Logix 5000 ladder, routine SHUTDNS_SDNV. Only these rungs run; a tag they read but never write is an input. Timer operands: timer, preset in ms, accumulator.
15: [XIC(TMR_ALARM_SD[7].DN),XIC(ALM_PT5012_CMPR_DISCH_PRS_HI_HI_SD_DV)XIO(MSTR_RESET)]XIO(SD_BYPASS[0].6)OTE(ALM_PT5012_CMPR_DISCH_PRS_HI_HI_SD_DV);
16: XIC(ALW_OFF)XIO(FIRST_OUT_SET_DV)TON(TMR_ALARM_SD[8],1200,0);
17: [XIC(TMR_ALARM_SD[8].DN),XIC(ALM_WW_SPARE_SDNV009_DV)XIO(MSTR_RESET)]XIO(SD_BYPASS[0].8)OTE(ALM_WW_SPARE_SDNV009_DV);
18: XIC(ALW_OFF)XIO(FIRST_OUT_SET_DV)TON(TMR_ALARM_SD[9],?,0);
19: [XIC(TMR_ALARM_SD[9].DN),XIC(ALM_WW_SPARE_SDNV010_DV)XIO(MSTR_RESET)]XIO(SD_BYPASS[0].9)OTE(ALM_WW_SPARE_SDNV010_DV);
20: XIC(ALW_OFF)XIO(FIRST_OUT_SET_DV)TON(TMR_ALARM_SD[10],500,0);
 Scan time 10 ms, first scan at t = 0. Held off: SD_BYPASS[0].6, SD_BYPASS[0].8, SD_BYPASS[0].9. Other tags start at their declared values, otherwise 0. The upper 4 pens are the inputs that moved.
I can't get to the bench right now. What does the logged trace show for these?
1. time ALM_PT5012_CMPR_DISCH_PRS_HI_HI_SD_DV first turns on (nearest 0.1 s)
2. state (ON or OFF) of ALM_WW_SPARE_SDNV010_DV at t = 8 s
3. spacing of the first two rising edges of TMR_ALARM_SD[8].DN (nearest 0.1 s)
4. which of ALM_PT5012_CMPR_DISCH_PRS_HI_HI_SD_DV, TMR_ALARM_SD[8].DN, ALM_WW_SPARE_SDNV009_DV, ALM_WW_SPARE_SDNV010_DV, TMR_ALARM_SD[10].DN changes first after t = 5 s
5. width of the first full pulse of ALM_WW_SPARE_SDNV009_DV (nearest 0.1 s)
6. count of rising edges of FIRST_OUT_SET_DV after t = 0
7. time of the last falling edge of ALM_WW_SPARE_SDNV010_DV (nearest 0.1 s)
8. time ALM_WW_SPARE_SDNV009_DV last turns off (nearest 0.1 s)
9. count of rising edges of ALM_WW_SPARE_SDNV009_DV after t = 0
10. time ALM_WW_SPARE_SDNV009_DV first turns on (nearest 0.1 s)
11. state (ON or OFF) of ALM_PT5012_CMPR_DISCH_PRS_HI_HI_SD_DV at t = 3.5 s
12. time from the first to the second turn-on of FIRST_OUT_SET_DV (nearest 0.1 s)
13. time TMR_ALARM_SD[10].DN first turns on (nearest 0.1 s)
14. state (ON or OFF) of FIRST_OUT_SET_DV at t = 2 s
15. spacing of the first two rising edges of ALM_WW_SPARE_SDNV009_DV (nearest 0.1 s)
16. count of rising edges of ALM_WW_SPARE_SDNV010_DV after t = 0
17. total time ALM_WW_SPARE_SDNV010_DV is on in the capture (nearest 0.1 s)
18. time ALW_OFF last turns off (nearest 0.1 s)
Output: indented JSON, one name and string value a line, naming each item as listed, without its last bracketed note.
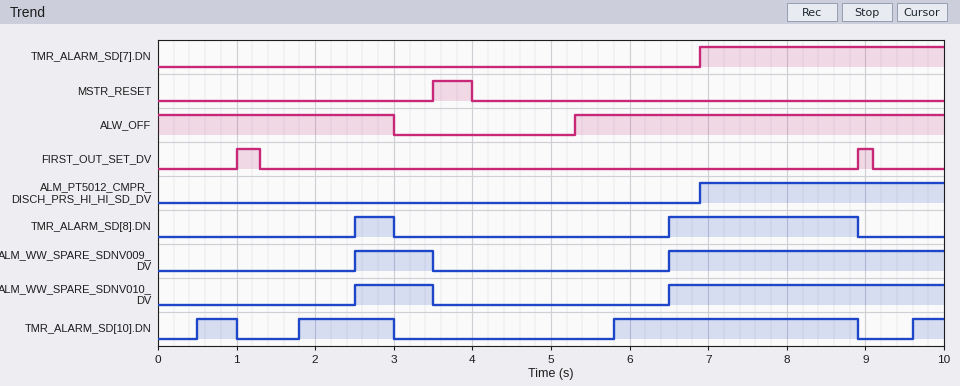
{
  "time ALM_PT5012_CMPR_DISCH_PRS_HI_HI_SD_DV first turns on": "6.9 s",
  "state (ON or OFF) of ALM_WW_SPARE_SDNV010_DV at t = 8 s": "ON",
  "spacing of the first two rising edges of TMR_ALARM_SD[8].DN": "4.0 s",
  "which of ALM_PT5012_CMPR_DISCH_PRS_HI_HI_SD_DV, TMR_ALARM_SD[8].DN, ALM_WW_SPARE_SDNV009_DV, ALM_WW_SPARE_SDNV010_DV, TMR_ALARM_SD[10].DN changes first after t = 5 s": "TMR_ALARM_SD[10].DN",
  "width of the first full pulse of ALM_WW_SPARE_SDNV009_DV": "1.0 s",
  "count of rising edges of FIRST_OUT_SET_DV after t = 0": "2",
  "time of the last falling edge of ALM_WW_SPARE_SDNV010_DV": "3.5 s",
  "time ALM_WW_SPARE_SDNV009_DV last turns off": "3.5 s",
  "count of rising edges of ALM_WW_SPARE_SDNV009_DV after t = 0": "2",
  "time ALM_WW_SPARE_SDNV009_DV first turns on": "2.5 s",
  "state (ON or OFF) of ALM_PT5012_CMPR_DISCH_PRS_HI_HI_SD_DV at t = 3.5 s": "OFF",
  "time from the first to the second turn-on of FIRST_OUT_SET_DV": "7.9 s",
  "time TMR_ALARM_SD[10].DN first turns on": "0.5 s",
  "state (ON or OFF) of FIRST_OUT_SET_DV at t = 2 s": "OFF",
  "spacing of the first two rising edges of ALM_WW_SPARE_SDNV009_DV": "4.0 s",
  "count of rising edges of ALM_WW_SPARE_SDNV010_DV after t = 0": "2",
  "total time ALM_WW_SPARE_SDNV010_DV is on in the capture": "4.5 s",
  "time ALW_OFF last turns off": "3.0 s"
}
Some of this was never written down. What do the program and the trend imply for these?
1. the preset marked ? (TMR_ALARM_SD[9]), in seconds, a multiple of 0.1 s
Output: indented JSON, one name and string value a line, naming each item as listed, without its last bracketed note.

{
  "the preset marked ? (TMR_ALARM_SD[9]), in seconds, a multiple of 0.1 s": "1.2 s"
}
